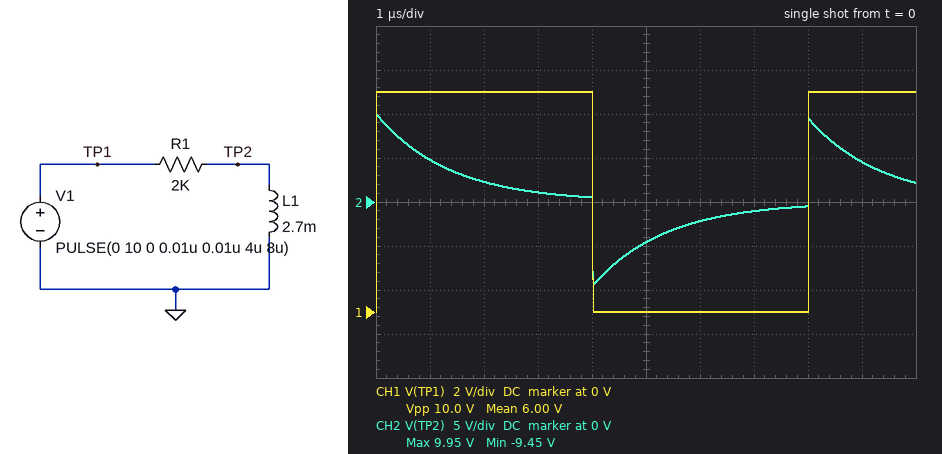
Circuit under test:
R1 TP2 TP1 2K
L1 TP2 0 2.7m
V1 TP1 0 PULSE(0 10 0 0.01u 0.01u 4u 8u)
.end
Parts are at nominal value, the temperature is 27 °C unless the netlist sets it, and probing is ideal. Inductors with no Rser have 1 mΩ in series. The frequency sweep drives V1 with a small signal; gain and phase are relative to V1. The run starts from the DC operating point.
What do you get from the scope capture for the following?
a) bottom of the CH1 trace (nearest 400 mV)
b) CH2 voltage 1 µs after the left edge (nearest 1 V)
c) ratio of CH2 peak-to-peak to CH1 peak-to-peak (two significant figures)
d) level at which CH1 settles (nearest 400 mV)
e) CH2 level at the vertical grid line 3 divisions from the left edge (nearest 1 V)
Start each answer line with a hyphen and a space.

- 0 V
- 5 V
- 1.9
- 10.0 V
- 1 V
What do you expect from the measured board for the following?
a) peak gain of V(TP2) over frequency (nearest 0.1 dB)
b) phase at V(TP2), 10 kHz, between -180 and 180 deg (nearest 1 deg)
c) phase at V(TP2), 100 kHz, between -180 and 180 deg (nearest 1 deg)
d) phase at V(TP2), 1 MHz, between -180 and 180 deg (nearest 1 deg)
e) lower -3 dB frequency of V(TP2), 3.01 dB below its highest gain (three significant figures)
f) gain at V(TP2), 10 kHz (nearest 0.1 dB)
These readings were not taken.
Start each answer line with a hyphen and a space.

- 0 dB
- 85 deg
- 50 deg
- 7 deg
- 118 kHz
- -21.5 dB
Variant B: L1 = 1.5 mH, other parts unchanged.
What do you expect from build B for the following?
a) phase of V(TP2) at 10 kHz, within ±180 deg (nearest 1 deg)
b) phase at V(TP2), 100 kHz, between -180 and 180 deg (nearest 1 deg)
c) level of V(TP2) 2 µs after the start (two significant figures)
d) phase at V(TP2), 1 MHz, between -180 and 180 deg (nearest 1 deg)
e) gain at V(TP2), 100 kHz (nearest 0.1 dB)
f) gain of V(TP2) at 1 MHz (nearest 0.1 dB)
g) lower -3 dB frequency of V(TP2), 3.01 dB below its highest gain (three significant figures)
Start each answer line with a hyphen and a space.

- 87 deg
- 65 deg
- 700 mV
- 12 deg
- -7.4 dB
- -0.2 dB
- 212 kHz
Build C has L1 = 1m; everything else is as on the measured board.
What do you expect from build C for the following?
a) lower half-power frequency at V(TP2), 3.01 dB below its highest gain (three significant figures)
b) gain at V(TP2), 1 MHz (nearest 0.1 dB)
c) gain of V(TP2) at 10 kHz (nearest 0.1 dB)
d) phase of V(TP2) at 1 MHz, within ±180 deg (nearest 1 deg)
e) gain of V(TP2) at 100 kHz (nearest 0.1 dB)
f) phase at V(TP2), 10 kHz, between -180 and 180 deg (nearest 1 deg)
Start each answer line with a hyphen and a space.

- 318 kHz
- -0.4 dB
- -30.1 dB
- 18 deg
- -10.5 dB
- 88 deg
